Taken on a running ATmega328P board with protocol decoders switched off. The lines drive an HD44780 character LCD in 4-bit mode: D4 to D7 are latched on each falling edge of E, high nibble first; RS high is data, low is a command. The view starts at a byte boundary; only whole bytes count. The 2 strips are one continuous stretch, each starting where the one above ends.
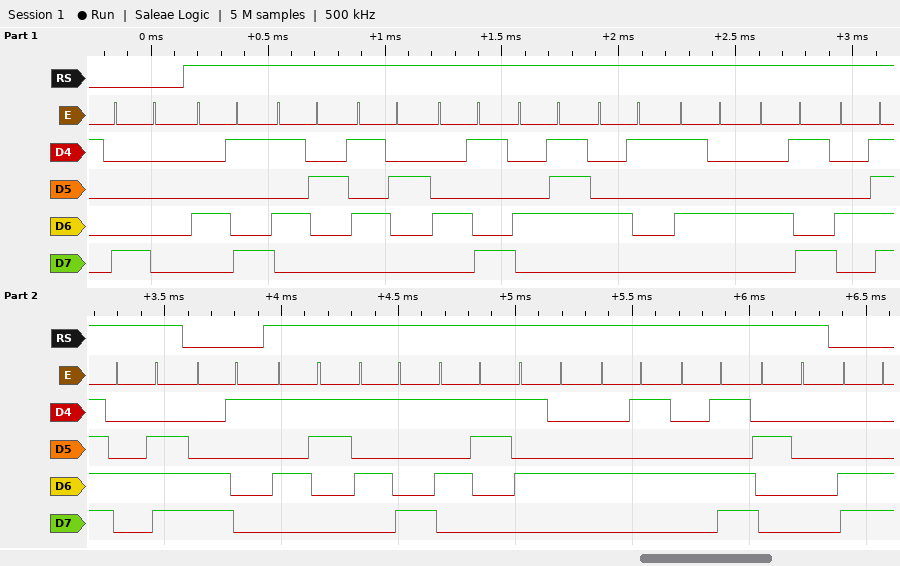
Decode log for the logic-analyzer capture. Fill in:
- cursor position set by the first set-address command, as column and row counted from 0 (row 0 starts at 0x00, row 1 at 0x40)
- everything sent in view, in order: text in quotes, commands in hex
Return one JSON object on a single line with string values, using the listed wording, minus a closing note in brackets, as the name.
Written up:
{"cursor position set by the first set-address command, as column and row counted from 0": "column 0, row 0", "everything sent in view, in order: text in quotes, commands in hex": "0x80 \"IRRIGATION\" 0xC1 \"SYSTEM \" 0xCC"}
